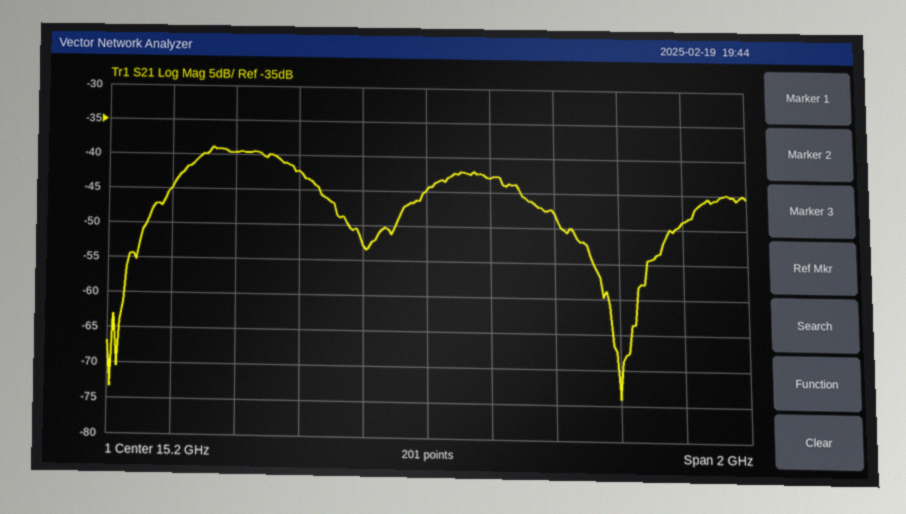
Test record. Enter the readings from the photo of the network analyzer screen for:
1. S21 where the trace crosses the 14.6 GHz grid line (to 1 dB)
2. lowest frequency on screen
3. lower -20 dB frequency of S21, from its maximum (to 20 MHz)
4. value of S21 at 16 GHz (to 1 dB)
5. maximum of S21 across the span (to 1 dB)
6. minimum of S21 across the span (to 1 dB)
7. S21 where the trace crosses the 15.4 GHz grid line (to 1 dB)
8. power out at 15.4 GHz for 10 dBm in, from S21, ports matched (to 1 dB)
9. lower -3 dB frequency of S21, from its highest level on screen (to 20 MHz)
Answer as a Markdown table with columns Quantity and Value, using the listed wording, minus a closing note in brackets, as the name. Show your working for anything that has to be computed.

| Quantity | Value |
|---|---|
| S21 where the trace crosses the 14.6 GHz grid line | -40 dB |
| lowest frequency on screen | 14.2 GHz |
| lower -20 dB frequency of S21, from its maximum | 14.26 GHz |
| value of S21 at 16 GHz | -49 dB |
| maximum of S21 across the span | -39 dB |
| minimum of S21 across the span | -74 dB |
| S21 where the trace crosses the 15.4 GHz grid line | -43 dB |
| power out at 15.4 GHz for 10 dBm in, from S21, ports matched | 10 dBm + (-43 dB) = -33 dBm |
| lower -3 dB frequency of S21, from its highest level on screen | 14.44 GHz |
